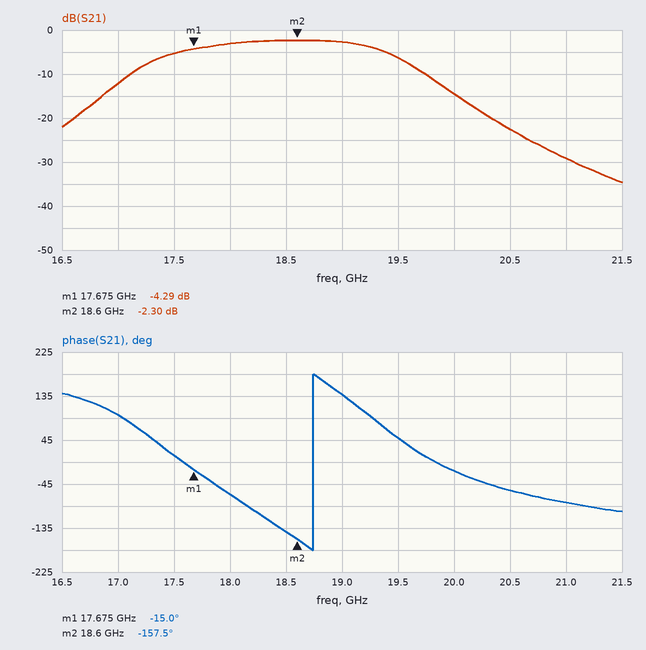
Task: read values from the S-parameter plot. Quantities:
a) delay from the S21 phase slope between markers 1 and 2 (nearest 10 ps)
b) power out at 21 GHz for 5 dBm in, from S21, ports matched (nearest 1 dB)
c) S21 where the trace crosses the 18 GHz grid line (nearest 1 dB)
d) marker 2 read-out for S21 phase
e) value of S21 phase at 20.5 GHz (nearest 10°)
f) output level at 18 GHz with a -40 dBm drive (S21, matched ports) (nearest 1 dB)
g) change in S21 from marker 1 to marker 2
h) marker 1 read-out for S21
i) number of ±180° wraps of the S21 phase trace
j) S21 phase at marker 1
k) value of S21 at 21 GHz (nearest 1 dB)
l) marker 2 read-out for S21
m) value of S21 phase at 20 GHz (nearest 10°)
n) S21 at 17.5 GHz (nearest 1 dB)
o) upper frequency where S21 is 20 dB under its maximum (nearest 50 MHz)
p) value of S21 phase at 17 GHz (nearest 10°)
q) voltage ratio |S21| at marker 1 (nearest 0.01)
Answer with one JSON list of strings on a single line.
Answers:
["430 ps", "-24 dBm", "-3 dB", "-157.5°", "-60°", "-43 dBm", "1.99 dB", "-4.29 dB", "1", "-15.0°", "-29 dB", "-2.30 dB", "-20°", "-5 dB", "20.50 GHz", "100°", "0.61"]
